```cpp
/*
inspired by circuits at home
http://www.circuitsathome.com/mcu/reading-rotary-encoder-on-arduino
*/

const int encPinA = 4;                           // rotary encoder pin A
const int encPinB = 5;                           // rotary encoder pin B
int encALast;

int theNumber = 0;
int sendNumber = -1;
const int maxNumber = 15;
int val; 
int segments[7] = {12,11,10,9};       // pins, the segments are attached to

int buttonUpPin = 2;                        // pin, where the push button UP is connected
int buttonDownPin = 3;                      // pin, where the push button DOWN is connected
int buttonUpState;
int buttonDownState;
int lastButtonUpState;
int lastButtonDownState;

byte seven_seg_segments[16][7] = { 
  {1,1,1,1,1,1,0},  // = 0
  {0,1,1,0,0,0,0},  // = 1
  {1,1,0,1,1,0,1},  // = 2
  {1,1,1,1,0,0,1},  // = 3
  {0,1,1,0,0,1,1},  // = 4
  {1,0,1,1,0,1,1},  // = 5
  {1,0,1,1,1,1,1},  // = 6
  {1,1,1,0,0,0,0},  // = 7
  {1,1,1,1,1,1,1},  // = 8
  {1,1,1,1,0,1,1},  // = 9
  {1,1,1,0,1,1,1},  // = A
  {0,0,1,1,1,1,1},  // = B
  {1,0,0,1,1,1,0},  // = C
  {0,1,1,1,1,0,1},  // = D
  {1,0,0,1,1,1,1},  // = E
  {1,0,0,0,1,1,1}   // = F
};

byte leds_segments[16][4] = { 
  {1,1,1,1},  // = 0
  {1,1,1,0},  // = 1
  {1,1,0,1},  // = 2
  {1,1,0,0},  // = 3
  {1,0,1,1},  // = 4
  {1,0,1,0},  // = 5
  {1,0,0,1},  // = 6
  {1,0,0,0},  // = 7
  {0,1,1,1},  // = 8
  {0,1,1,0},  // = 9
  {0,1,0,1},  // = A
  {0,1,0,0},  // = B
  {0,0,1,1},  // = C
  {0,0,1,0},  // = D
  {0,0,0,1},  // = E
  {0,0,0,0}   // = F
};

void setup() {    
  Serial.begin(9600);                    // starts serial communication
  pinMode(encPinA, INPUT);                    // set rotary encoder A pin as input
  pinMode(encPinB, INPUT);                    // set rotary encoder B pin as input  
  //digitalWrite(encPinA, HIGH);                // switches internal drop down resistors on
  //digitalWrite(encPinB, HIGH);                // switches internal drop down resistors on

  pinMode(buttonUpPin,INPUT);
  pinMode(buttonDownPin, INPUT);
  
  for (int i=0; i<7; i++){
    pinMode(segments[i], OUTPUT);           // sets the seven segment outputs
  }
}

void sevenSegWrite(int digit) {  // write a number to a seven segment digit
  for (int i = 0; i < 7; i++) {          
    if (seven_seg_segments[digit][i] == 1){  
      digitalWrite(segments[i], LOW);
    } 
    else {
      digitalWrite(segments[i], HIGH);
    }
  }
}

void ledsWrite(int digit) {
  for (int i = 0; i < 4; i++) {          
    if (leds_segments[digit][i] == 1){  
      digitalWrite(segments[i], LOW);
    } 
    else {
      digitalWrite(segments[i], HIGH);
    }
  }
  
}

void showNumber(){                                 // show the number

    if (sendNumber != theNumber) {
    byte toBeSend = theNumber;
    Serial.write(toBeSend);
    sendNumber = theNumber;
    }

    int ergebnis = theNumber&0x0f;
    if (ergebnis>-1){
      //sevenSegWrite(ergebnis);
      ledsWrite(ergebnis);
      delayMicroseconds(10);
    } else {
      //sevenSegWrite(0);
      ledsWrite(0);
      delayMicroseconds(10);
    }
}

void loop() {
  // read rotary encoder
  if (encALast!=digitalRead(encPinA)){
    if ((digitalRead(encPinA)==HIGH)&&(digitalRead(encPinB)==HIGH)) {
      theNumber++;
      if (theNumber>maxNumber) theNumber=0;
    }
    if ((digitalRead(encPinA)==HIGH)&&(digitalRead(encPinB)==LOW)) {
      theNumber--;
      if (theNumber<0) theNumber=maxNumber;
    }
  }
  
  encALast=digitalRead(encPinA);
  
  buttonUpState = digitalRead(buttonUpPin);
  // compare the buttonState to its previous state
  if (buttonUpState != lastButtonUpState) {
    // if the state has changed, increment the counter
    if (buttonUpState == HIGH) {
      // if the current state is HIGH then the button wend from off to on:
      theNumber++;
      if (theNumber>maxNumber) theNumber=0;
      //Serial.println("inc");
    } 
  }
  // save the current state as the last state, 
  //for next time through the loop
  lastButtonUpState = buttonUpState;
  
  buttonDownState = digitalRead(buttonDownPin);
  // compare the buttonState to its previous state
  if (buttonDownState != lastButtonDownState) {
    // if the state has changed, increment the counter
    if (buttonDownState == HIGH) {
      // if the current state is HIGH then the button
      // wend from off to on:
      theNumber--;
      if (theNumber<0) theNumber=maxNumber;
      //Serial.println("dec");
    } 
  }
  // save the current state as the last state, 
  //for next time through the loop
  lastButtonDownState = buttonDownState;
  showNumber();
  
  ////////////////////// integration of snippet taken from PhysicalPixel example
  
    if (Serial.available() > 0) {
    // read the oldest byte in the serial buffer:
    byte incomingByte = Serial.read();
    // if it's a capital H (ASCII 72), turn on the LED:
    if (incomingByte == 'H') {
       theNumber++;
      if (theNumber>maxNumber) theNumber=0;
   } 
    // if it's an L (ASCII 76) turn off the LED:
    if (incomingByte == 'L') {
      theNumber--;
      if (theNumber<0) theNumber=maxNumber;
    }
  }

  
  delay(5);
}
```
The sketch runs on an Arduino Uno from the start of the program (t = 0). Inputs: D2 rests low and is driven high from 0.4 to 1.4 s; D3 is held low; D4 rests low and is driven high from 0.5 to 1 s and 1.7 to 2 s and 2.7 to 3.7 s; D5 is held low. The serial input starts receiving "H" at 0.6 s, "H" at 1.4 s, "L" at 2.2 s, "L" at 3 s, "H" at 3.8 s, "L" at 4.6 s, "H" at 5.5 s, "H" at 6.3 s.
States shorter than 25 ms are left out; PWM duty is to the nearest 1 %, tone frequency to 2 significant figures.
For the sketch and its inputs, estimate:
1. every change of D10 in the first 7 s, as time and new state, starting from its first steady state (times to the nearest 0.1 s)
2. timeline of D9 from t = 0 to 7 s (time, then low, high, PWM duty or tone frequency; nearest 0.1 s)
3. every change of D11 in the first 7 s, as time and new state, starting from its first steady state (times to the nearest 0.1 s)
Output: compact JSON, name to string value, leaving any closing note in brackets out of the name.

{"every change of D10 in the first 7 s, as time and new state, starting from its first steady state": "0 s low; 1.4 s high; 1.7 s low; 2.7 s high; 6.3 s low", "timeline of D9 from t = 0 to 7 s": "0 s low; 0.4 s high; 0.5 s low; 0.6 s high; 1.4 s low; 1.7 s high; 2.2 s low; 2.7 s high; 3 s low; 3.8 s high; 4.6 s low; 5.5 s high; 6.3 s low", "every change of D11 in the first 7 s, as time and new state, starting from its first steady state": "0 s low; 2.7 s high; 6.3 s low"}
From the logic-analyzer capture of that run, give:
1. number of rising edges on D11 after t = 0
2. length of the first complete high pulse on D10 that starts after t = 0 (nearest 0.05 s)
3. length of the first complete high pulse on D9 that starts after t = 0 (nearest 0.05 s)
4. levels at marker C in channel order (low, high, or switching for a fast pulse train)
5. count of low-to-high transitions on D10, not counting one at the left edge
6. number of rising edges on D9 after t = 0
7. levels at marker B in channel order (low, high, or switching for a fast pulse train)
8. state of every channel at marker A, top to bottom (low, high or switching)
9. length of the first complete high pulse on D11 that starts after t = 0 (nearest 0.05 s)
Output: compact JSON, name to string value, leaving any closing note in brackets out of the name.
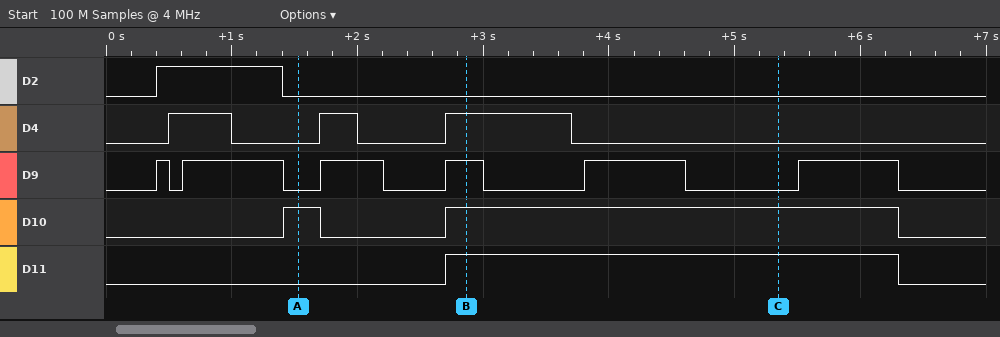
{"number of rising edges on D11 after t = 0": "1", "length of the first complete high pulse on D10 that starts after t = 0": "0.30 s", "length of the first complete high pulse on D9 that starts after t = 0": "0.10 s", "levels at marker C in channel order": "D2 low, D4 low, D9 low, D10 high, D11 high", "count of low-to-high transitions on D10, not counting one at the left edge": "2", "number of rising edges on D9 after t = 0": "6", "levels at marker B in channel order": "D2 low, D4 high, D9 high, D10 high, D11 high", "state of every channel at marker A, top to bottom": "D2 low, D4 low, D9 low, D10 high, D11 low", "length of the first complete high pulse on D11 that starts after t = 0": "3.60 s"}
